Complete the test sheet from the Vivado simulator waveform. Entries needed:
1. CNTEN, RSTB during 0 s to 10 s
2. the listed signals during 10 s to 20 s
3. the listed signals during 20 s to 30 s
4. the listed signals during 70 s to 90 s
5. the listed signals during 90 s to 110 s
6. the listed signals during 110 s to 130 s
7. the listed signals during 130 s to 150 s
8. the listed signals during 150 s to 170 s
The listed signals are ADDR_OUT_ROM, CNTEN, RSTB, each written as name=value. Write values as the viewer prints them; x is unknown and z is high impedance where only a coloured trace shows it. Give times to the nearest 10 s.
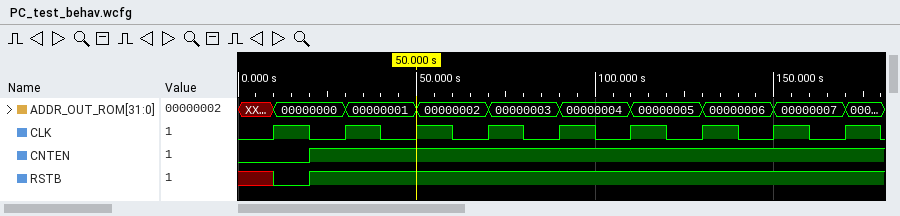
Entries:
CNTEN=0, RSTB=x
ADDR_OUT_ROM=00000000, CNTEN=0, RSTB=0
ADDR_OUT_ROM=00000000, CNTEN=1, RSTB=1
ADDR_OUT_ROM=00000003, CNTEN=1, RSTB=1
ADDR_OUT_ROM=00000004, CNTEN=1, RSTB=1
ADDR_OUT_ROM=00000005, CNTEN=1, RSTB=1
ADDR_OUT_ROM=00000006, CNTEN=1, RSTB=1
ADDR_OUT_ROM=00000007, CNTEN=1, RSTB=1
